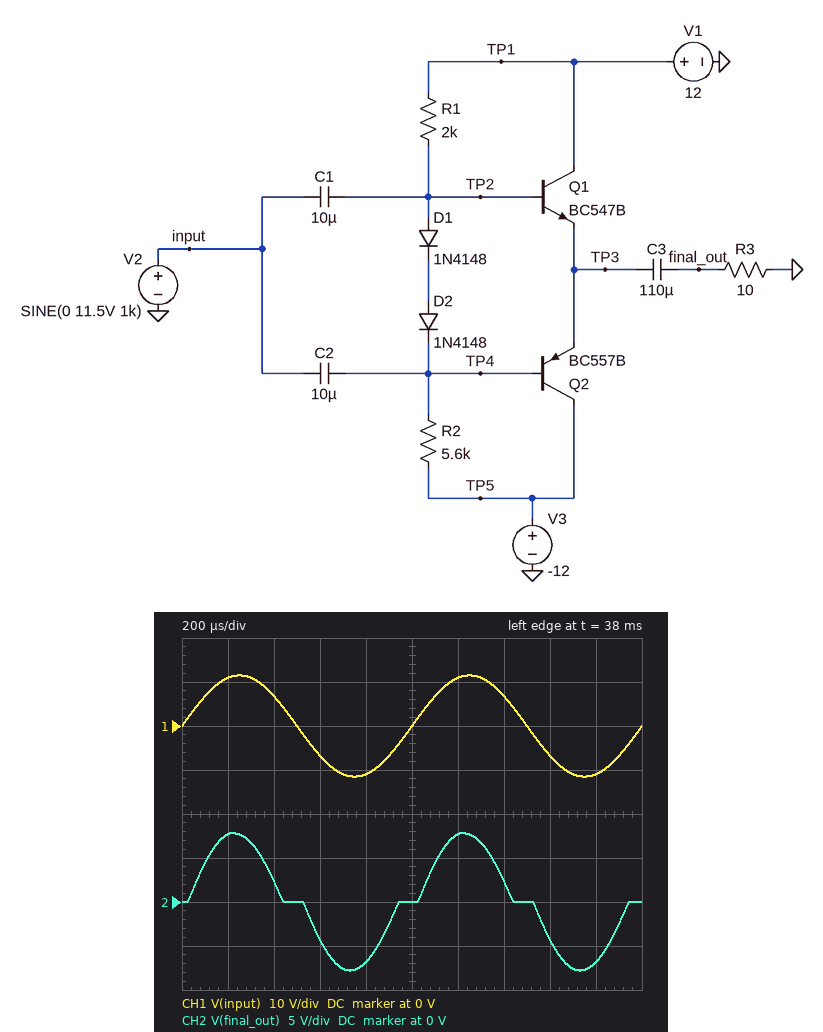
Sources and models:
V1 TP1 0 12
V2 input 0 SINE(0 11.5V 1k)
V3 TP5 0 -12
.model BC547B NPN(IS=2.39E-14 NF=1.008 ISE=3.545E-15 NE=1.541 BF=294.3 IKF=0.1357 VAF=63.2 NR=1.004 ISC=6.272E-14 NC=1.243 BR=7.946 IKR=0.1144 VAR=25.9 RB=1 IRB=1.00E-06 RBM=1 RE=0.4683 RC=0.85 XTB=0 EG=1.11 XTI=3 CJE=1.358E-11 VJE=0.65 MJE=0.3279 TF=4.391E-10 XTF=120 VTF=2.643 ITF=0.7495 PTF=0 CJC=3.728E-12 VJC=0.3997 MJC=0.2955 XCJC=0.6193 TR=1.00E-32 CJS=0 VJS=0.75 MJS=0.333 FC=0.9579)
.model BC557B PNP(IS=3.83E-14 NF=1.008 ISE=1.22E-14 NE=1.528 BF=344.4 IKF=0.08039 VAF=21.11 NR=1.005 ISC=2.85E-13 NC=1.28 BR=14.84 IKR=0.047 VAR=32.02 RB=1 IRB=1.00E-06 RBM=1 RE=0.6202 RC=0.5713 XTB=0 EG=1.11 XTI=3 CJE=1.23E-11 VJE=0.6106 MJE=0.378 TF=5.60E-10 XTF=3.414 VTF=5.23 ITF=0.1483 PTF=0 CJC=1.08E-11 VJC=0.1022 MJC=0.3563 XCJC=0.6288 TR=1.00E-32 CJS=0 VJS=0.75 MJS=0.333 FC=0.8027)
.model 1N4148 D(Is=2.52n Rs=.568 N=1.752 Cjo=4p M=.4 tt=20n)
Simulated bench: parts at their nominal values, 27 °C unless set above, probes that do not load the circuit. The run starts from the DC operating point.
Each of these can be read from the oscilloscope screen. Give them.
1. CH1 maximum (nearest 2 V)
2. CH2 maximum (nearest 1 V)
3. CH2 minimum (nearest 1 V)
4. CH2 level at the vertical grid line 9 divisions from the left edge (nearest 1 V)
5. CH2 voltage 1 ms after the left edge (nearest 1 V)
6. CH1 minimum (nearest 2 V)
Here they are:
12 V
8 V
-8 V
-7 V
0 V
-12 V
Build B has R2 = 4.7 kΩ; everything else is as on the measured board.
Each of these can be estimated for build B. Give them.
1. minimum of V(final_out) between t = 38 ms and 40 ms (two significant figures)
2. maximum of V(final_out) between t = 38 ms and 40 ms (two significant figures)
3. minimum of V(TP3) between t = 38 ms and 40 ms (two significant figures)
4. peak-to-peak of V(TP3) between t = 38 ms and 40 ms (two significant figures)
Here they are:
-8.1 V
8.1 V
-5.4 V
16 V
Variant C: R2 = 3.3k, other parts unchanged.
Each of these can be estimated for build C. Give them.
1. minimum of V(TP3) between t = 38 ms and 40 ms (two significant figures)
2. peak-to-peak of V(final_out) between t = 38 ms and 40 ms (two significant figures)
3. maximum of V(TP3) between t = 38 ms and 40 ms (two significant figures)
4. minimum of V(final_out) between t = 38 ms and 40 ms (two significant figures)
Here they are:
-6.7 V
17 V
11 V
-8.7 V
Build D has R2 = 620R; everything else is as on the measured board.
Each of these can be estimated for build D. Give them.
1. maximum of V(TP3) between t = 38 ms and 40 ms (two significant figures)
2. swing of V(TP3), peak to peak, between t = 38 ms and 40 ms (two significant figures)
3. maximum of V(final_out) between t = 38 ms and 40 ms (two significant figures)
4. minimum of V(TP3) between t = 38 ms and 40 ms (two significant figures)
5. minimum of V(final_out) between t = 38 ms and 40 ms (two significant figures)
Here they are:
8.8 V
20 V
10 V
-11 V
-9.9 V
